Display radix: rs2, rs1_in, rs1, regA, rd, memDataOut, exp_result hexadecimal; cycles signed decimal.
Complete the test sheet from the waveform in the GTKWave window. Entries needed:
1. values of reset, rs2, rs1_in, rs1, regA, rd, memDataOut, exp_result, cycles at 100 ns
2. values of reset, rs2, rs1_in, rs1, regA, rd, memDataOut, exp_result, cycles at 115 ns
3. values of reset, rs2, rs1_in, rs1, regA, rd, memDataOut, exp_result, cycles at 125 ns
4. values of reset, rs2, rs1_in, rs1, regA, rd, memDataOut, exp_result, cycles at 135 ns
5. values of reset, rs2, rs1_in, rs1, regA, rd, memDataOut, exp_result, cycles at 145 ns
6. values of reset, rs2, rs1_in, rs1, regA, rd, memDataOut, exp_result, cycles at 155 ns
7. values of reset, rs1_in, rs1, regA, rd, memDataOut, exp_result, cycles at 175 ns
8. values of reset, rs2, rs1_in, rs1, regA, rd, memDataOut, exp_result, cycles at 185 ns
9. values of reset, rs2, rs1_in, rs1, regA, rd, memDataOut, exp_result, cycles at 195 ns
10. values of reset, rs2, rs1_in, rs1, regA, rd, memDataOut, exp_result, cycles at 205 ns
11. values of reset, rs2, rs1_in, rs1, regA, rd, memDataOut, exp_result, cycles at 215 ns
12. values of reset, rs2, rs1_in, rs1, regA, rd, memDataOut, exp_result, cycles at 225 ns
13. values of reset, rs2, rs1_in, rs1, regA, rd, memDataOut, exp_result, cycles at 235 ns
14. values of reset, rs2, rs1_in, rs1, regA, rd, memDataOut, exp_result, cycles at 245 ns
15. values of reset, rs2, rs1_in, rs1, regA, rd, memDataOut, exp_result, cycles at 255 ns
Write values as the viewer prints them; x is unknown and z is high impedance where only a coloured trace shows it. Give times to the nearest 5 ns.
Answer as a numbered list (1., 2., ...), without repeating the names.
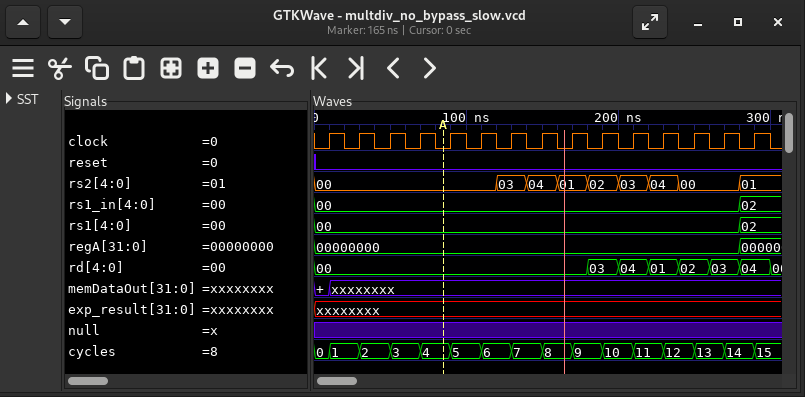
1. reset=0, rs2=00, rs1_in=00, rs1=00, regA=00000000, rd=00, memDataOut=xxxxxxxx, exp_result=xxxxxxxx, cycles=5
2. reset=0, rs2=00, rs1_in=00, rs1=00, regA=00000000, rd=00, memDataOut=xxxxxxxx, exp_result=xxxxxxxx, cycles=6
3. reset=0, rs2=03, rs1_in=00, rs1=00, regA=00000000, rd=00, memDataOut=xxxxxxxx, exp_result=xxxxxxxx, cycles=6
4. reset=0, rs2=03, rs1_in=00, rs1=00, regA=00000000, rd=00, memDataOut=xxxxxxxx, exp_result=xxxxxxxx, cycles=7
5. reset=0, rs2=04, rs1_in=00, rs1=00, regA=00000000, rd=00, memDataOut=xxxxxxxx, exp_result=xxxxxxxx, cycles=7
6. reset=0, rs2=04, rs1_in=00, rs1=00, regA=00000000, rd=00, memDataOut=xxxxxxxx, exp_result=xxxxxxxx, cycles=8
7. reset=0, rs1_in=00, rs1=00, regA=00000000, rd=00, memDataOut=xxxxxxxx, exp_result=xxxxxxxx, cycles=9
8. reset=0, rs2=02, rs1_in=00, rs1=00, regA=00000000, rd=03, memDataOut=xxxxxxxx, exp_result=xxxxxxxx, cycles=9
9. reset=0, rs2=02, rs1_in=00, rs1=00, regA=00000000, rd=03, memDataOut=xxxxxxxx, exp_result=xxxxxxxx, cycles=10
10. reset=0, rs2=03, rs1_in=00, rs1=00, regA=00000000, rd=04, memDataOut=xxxxxxxx, exp_result=xxxxxxxx, cycles=10
11. reset=0, rs2=03, rs1_in=00, rs1=00, regA=00000000, rd=04, memDataOut=xxxxxxxx, exp_result=xxxxxxxx, cycles=11
12. reset=0, rs2=04, rs1_in=00, rs1=00, regA=00000000, rd=01, memDataOut=xxxxxxxx, exp_result=xxxxxxxx, cycles=11
13. reset=0, rs2=04, rs1_in=00, rs1=00, regA=00000000, rd=01, memDataOut=xxxxxxxx, exp_result=xxxxxxxx, cycles=12
14. reset=0, rs2=00, rs1_in=00, rs1=00, regA=00000000, rd=02, memDataOut=xxxxxxxx, exp_result=xxxxxxxx, cycles=12
15. reset=0, rs2=00, rs1_in=00, rs1=00, regA=00000000, rd=02, memDataOut=xxxxxxxx, exp_result=xxxxxxxx, cycles=13
